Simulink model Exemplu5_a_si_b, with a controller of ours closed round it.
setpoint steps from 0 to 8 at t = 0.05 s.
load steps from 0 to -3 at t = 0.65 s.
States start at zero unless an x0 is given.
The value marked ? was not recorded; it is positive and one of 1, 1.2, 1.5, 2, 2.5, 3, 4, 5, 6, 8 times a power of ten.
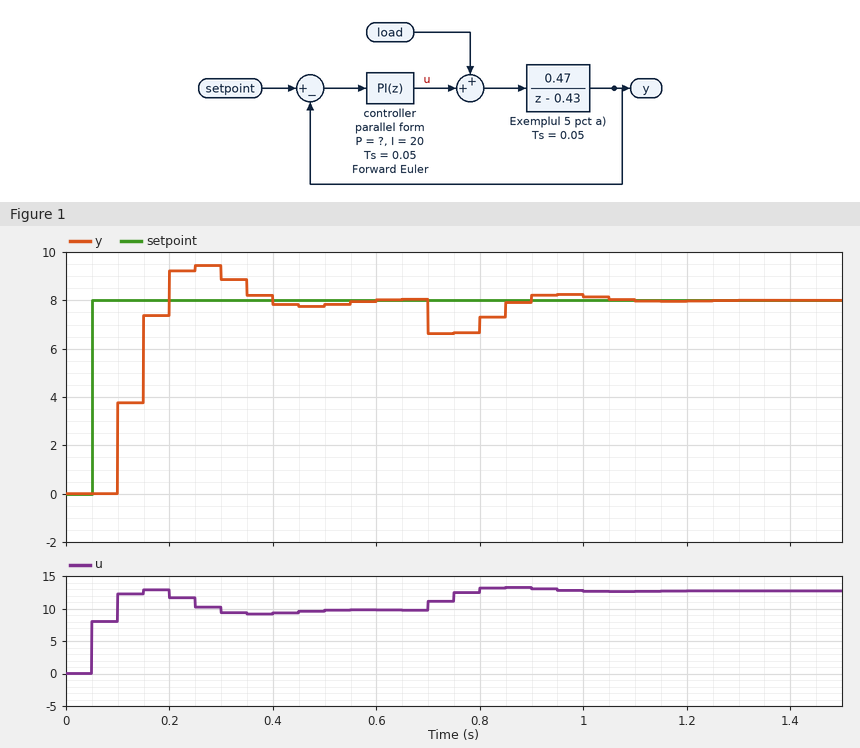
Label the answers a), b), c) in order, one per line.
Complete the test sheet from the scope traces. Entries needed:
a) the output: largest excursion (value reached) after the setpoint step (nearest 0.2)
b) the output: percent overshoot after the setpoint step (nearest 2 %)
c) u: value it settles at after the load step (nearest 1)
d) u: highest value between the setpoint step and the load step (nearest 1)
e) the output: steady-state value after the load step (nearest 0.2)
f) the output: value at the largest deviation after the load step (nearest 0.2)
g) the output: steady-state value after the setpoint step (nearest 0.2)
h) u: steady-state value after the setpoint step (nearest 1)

a) 9.4
b) 18 %
c) 13
d) 13
e) 8.0
f) 6.6
g) 8.0
h) 10
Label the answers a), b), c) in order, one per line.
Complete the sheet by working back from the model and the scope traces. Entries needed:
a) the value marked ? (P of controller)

a) 1
